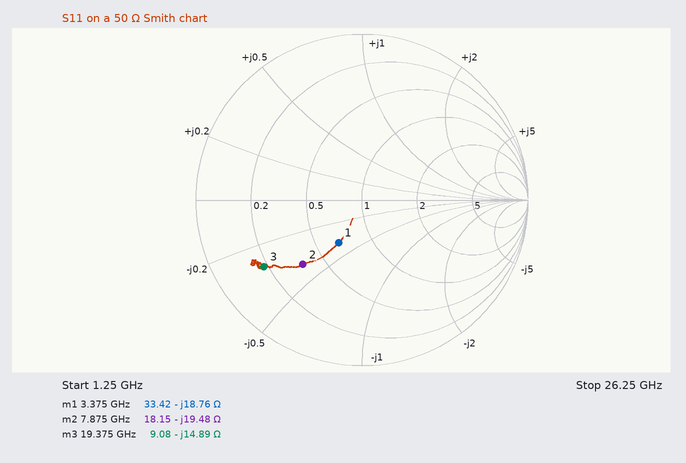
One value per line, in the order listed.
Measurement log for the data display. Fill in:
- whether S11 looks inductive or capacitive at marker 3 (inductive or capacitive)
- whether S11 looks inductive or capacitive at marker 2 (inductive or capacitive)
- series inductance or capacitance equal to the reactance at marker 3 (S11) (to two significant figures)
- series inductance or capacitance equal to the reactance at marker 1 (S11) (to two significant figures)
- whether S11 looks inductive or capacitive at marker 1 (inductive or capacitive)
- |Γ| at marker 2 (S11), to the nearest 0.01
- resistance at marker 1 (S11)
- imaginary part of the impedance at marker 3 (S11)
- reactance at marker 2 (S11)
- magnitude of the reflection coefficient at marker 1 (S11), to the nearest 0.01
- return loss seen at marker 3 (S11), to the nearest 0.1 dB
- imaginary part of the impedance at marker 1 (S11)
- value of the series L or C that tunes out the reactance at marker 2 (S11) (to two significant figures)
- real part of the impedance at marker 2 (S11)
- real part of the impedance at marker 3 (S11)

capacitive
capacitive
550 fF
2.5 pF
capacitive
0.53
33.42 Ω
-14.89 Ω
-19.48 Ω
0.29
2.9 dB
-18.76 Ω
390 pH
18.15 Ω
9.08 Ω
